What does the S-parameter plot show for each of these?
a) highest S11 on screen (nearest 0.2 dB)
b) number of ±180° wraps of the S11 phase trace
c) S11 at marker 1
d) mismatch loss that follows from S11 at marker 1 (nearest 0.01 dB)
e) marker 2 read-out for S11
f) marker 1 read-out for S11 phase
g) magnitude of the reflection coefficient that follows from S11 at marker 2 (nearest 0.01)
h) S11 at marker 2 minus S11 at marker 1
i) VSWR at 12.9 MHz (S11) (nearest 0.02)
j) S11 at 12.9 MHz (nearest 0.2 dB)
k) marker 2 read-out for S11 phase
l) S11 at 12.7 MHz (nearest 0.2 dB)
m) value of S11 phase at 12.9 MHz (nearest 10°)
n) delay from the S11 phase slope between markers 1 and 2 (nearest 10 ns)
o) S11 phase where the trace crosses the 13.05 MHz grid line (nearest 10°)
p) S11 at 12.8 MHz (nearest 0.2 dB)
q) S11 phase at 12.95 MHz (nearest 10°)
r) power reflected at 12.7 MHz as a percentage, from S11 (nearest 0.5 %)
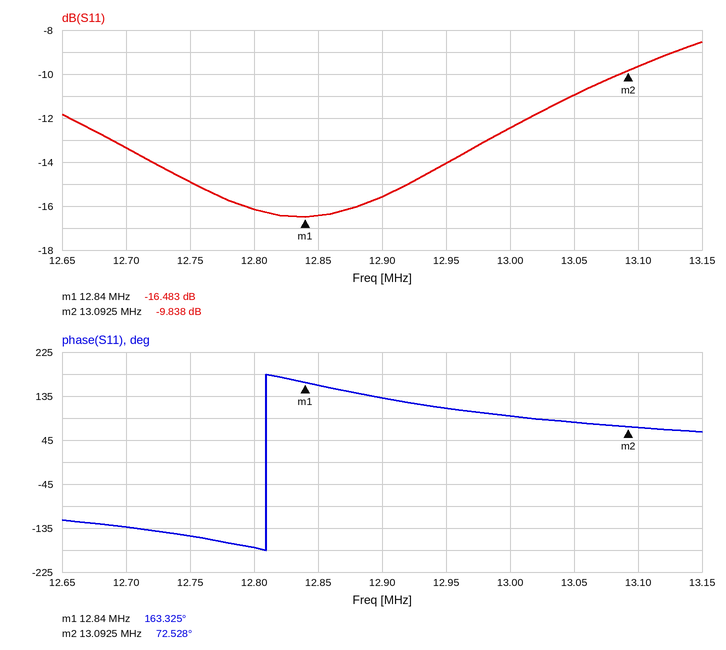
-8.6 dB
1
-16.483 dB
0.10 dB
-9.838 dB
163.325°
0.32
6.645 dB
1.40
-15.6 dB
72.528°
-13.4 dB
130°
1.00 µs
80°
-16.2 dB
110°
4.5 %
